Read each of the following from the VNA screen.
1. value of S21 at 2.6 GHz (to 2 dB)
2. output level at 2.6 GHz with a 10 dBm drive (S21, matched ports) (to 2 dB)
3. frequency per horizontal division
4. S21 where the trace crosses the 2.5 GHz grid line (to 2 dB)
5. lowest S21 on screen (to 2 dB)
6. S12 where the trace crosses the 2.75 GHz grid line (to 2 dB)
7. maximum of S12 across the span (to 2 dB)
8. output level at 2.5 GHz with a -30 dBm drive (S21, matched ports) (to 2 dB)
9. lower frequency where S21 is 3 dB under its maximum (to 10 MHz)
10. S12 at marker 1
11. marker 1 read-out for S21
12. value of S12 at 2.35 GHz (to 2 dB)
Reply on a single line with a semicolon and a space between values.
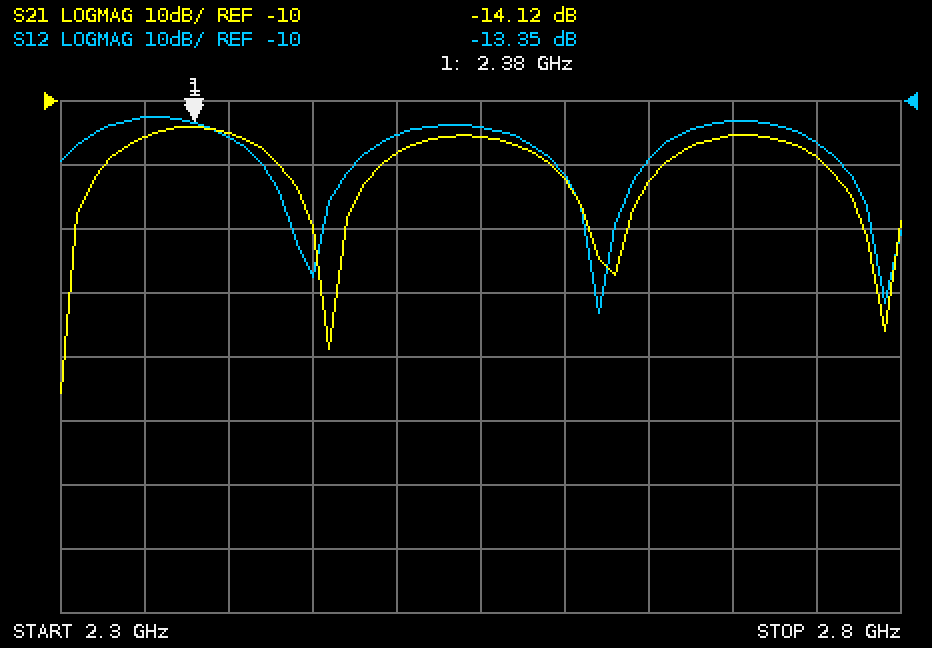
-22 dB; -12 dBm; 50 MHz; -18 dB; -56 dB; -16 dB; -12 dB; -48 dBm; 2.34 GHz; -13.35 dB; -14.12 dB; -12 dB
